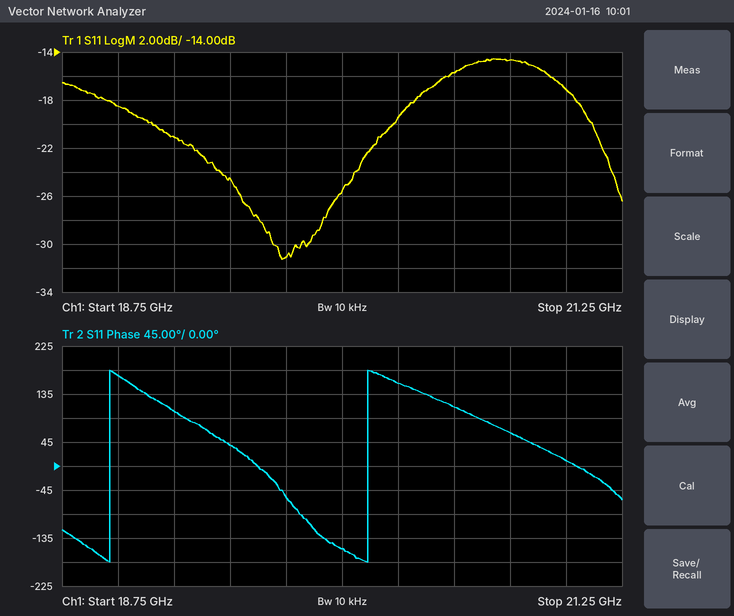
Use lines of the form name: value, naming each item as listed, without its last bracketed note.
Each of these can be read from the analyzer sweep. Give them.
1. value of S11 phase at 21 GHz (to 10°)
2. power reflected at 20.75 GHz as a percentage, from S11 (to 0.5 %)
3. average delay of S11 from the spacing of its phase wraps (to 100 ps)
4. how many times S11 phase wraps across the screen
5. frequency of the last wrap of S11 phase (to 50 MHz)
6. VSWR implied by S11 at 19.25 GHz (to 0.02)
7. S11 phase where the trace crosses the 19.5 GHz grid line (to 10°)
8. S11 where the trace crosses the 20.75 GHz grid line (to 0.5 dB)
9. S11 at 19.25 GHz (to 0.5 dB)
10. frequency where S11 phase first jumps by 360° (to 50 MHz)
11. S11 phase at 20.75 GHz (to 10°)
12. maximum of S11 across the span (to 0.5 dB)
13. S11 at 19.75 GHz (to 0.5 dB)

value of S11 phase at 21 GHz: 10°
power reflected at 20.75 GHz as a percentage, from S11: 3.5 %
average delay of S11 from the spacing of its phase wraps: 900 ps
how many times S11 phase wraps across the screen: 2
frequency of the last wrap of S11 phase: 20.10 GHz
VSWR implied by S11 at 19.25 GHz: 1.20
S11 phase where the trace crosses the 19.5 GHz grid line: 40°
S11 where the trace crosses the 20.75 GHz grid line: -14.5 dB
S11 at 19.25 GHz: -21.0 dB
frequency where S11 phase first jumps by 360°: 18.95 GHz
S11 phase at 20.75 GHz: 60°
maximum of S11 across the span: -14.5 dB
S11 at 19.75 GHz: -31.0 dB
